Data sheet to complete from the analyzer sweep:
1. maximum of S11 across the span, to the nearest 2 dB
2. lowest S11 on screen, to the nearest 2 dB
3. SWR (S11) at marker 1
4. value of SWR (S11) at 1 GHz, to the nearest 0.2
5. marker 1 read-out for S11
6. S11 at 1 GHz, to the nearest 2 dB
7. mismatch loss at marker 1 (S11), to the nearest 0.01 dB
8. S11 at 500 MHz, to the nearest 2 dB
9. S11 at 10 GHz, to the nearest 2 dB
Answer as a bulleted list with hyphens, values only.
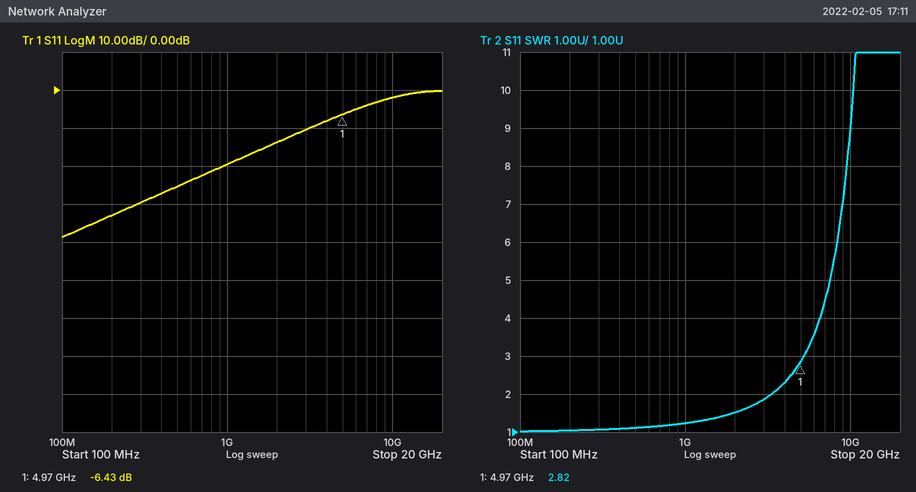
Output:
- 0 dB
- -38 dB
- 2.82
- 1.2
- -6.43 dB
- -20 dB
- 1.12 dB
- -26 dB
- -2 dB
